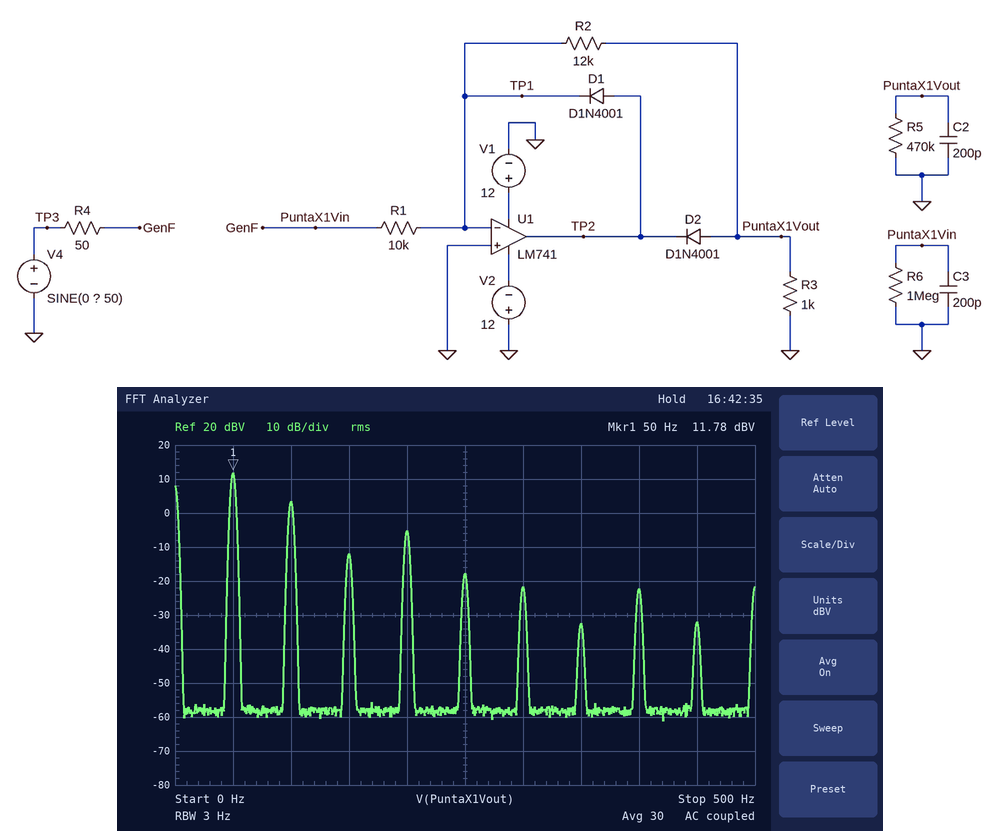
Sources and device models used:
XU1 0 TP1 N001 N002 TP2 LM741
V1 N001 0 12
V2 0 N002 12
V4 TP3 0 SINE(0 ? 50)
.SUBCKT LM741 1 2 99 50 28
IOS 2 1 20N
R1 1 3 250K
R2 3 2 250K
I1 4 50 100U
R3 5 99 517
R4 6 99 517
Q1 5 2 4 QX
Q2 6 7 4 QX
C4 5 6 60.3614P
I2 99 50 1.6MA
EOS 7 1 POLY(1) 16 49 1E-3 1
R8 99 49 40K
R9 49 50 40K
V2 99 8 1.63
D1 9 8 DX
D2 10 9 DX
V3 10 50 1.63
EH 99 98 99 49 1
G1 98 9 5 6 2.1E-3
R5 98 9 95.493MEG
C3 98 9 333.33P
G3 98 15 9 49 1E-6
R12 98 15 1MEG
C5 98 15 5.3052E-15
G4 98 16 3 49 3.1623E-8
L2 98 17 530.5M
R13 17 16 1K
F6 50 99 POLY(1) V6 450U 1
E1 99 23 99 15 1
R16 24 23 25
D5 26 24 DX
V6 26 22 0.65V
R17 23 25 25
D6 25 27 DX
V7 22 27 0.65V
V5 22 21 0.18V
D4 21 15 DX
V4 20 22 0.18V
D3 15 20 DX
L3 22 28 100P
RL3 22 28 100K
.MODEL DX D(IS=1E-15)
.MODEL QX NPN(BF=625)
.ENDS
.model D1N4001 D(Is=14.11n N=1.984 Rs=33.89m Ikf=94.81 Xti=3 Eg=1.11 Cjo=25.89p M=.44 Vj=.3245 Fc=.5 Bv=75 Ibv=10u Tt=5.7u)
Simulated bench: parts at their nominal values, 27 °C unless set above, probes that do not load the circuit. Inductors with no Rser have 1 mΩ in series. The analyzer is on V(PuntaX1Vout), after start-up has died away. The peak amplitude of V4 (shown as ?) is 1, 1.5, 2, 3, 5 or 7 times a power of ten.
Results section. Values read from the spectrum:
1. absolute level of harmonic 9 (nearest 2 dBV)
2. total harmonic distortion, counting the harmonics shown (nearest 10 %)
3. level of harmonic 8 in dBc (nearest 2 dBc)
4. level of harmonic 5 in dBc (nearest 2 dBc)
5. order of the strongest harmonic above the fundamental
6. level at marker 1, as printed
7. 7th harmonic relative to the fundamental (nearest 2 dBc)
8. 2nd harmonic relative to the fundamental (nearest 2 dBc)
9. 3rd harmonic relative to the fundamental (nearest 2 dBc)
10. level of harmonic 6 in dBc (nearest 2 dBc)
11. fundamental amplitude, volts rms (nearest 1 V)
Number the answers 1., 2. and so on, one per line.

1. -32 dBV
2. 40 %
3. -34 dBc
4. -30 dBc
5. 2
6. 11.78 dBV
7. -44 dBc
8. -8 dBc
9. -24 dBc
10. -34 dBc
11. 4 V
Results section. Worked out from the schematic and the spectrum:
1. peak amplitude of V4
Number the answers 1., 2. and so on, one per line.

1. 10 V
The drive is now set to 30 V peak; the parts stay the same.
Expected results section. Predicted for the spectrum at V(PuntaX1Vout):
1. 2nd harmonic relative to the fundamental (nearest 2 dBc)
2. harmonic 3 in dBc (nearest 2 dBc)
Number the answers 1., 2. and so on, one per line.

1. -18 dBc
2. -10 dBc
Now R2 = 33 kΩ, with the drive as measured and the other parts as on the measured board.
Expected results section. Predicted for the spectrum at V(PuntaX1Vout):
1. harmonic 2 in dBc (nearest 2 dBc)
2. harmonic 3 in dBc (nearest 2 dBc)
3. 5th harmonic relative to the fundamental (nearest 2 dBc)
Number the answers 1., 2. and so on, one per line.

1. -16 dBc
2. -10 dBc
3. -18 dBc
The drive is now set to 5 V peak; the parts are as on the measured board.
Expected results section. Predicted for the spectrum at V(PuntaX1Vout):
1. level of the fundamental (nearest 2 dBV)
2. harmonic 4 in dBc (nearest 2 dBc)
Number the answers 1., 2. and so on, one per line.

1. 6 dBV
2. -22 dBc
